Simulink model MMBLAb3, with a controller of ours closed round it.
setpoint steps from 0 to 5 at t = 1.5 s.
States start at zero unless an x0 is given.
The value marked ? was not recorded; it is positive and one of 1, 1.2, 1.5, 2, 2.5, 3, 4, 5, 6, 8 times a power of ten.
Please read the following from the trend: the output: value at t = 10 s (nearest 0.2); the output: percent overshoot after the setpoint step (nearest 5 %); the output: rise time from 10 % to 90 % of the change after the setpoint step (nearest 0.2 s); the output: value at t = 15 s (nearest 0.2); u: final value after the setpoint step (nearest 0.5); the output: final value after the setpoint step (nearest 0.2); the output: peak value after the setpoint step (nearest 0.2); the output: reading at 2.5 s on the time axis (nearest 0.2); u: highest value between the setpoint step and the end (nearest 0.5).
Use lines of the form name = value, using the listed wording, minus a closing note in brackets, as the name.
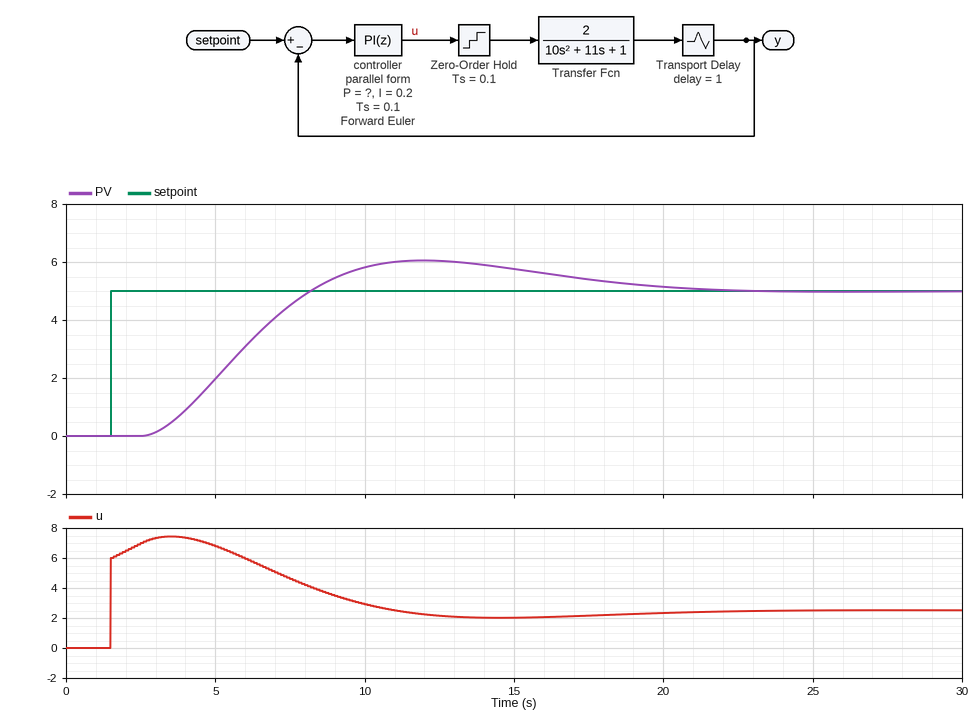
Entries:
the output: value at t = 10 s = 5.8
the output: percent overshoot after the setpoint step = 20 %
the output: rise time from 10 % to 90 % of the change after the setpoint step = 4.0 s
the output: value at t = 15 s = 5.8
u: final value after the setpoint step = 2.5
the output: final value after the setpoint step = 5.0
the output: peak value after the setpoint step = 6.0
the output: reading at 2.5 s on the time axis = 0.0
u: highest value between the setpoint step and the end = 7.5
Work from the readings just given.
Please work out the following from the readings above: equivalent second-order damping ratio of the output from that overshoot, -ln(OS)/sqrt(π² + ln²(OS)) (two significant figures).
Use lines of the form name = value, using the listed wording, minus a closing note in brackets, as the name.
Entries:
equivalent second-order damping ratio of the output from that overshoot, -ln(OS)/sqrt(π² + ln²(OS)) = 0.46
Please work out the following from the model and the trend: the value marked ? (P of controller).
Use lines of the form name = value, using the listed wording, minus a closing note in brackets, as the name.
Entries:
the value marked ? = 1.2
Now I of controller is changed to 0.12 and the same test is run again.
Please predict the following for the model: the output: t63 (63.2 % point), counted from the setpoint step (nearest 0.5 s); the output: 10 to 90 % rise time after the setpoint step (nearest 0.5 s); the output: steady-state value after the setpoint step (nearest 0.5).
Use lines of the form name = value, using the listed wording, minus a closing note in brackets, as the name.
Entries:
the output: t63 (63.2 % point), counted from the setpoint step = 5.0 s
the output: 10 to 90 % rise time after the setpoint step = 5.0 s
the output: steady-state value after the setpoint step = 5.0
